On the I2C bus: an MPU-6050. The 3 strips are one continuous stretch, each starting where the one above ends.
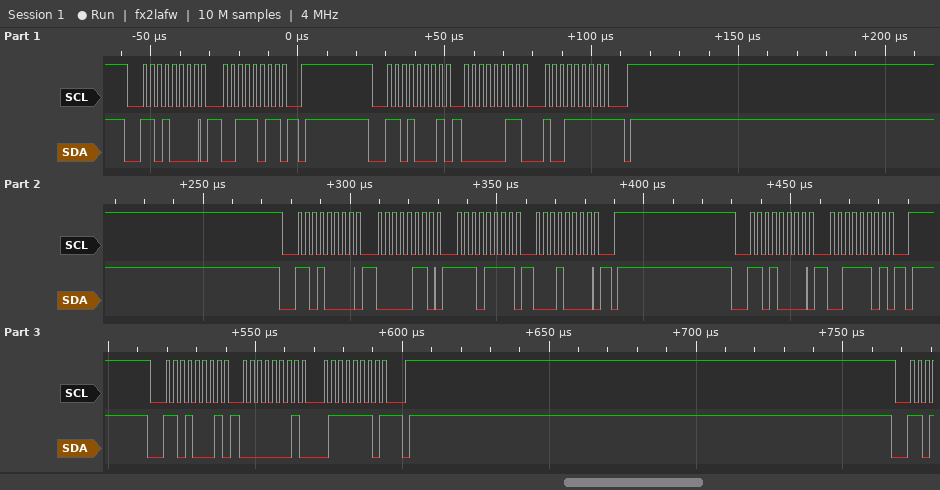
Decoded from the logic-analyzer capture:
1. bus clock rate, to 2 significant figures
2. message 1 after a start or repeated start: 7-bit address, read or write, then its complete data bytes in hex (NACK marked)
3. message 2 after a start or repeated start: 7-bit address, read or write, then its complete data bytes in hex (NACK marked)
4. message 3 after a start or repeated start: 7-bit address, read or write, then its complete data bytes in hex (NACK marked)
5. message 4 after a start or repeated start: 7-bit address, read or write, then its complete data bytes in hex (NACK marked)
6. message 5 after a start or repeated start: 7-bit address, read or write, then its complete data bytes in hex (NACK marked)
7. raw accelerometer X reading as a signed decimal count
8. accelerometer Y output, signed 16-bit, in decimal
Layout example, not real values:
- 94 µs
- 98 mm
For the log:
- 400 kHz
- 0x68 write: 3B
- 0x68 read: 03 9F NACK
- 0x68 write: 06 EF 10
- 0x68 write: 3D
- 0x68 read: 01 7E NACK
- 927
- 382
